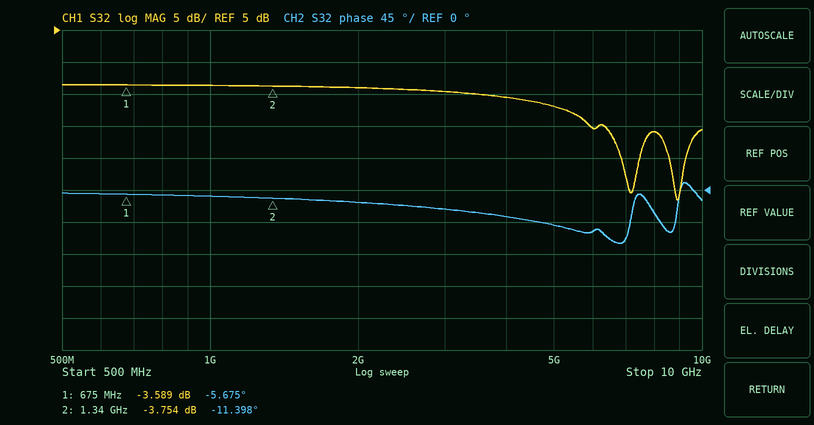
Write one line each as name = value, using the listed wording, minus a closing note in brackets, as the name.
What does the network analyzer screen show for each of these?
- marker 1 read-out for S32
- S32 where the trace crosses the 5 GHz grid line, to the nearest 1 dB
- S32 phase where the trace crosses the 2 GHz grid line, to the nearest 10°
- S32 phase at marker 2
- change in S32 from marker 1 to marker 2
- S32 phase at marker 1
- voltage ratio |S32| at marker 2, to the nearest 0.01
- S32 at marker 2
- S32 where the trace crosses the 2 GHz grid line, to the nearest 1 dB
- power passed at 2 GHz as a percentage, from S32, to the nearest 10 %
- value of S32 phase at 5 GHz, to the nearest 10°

marker 1 read-out for S32 = -3.589 dB
S32 where the trace crosses the 5 GHz grid line, to the nearest 1 dB = -7 dB
S32 phase where the trace crosses the 2 GHz grid line, to the nearest 10° = -20°
S32 phase at marker 2 = -11.398°
change in S32 from marker 1 to marker 2 = -0.165 dB
S32 phase at marker 1 = -5.675°
voltage ratio |S32| at marker 2, to the nearest 0.01 = 0.65
S32 at marker 2 = -3.754 dB
S32 where the trace crosses the 2 GHz grid line, to the nearest 1 dB = -4 dB
power passed at 2 GHz as a percentage, from S32, to the nearest 10 % = 40 %
value of S32 phase at 5 GHz, to the nearest 10° = -50°
